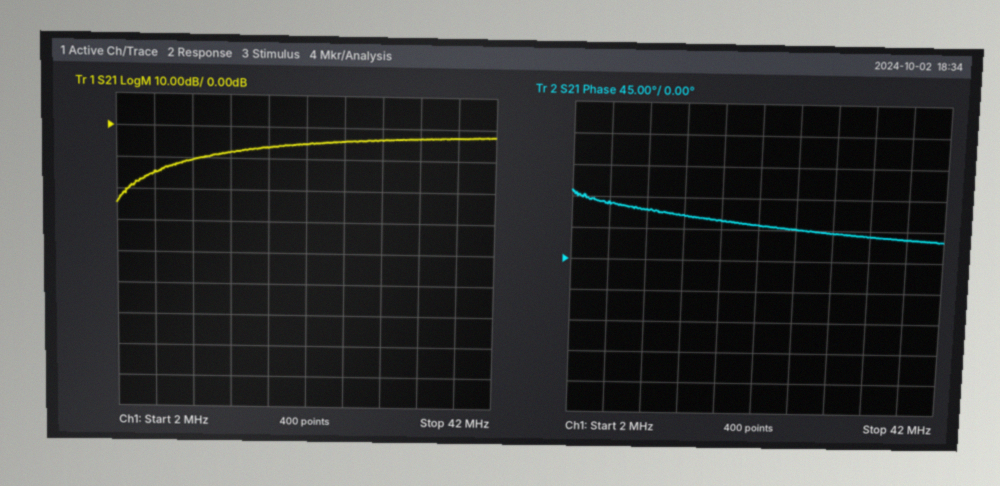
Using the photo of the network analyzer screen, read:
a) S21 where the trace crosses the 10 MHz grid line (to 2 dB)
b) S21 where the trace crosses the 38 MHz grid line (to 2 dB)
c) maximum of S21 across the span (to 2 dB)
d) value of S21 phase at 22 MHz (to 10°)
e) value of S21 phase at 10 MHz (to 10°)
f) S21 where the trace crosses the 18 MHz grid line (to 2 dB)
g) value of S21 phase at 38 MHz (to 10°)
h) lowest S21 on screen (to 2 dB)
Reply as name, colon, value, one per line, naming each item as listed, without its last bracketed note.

S21 where the trace crosses the 10 MHz grid line: -10 dB
S21 where the trace crosses the 38 MHz grid line: -2 dB
maximum of S21 across the span: -2 dB
value of S21 phase at 22 MHz: 50°
value of S21 phase at 10 MHz: 70°
S21 where the trace crosses the 18 MHz grid line: -6 dB
value of S21 phase at 38 MHz: 30°
lowest S21 on screen: -24 dB
